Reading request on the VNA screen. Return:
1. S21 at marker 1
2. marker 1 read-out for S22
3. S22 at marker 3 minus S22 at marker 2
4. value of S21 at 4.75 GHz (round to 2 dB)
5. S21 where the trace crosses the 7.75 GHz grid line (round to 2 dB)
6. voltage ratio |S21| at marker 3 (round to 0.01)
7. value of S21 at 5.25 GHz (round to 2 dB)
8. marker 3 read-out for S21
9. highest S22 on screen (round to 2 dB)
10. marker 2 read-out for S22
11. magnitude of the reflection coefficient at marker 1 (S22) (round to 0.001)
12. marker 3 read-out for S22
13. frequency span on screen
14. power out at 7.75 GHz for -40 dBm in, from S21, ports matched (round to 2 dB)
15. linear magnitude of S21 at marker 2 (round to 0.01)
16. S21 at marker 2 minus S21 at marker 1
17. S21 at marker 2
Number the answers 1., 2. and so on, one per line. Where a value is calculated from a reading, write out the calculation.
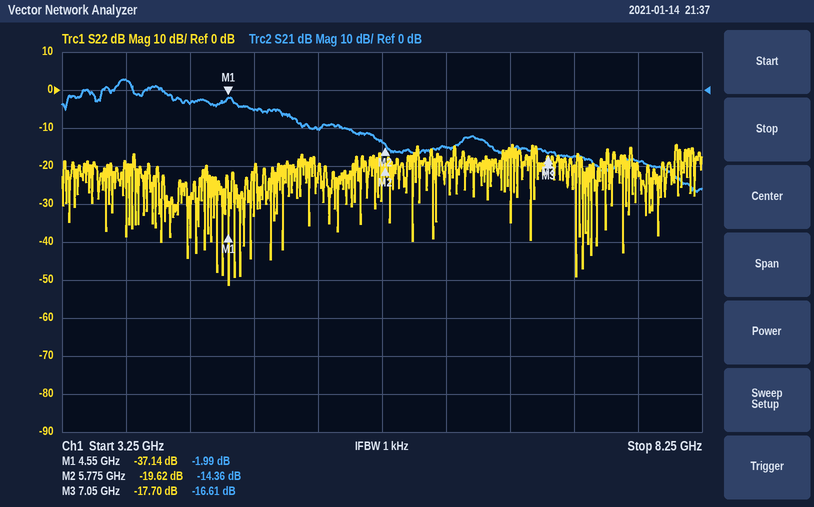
1. -1.99 dB
2. -37.14 dB
3. -17.7 − (-19.62) = 1.92 dB
4. -6 dB
5. -18 dB
6. 10^(-16.61/20) ≈ 0.15
7. -10 dB
8. -16.61 dB
9. -14 dB
10. -19.62 dB
11. 10^(-37.14/20) ≈ 0.014
12. -17.70 dB
13. 5 GHz
14. -40 dBm + (-18 dB) = -58 dBm
15. 10^(-14.36/20) ≈ 0.19
16. -14.36 − (-1.99) = -12.37 dB
17. -14.36 dB
